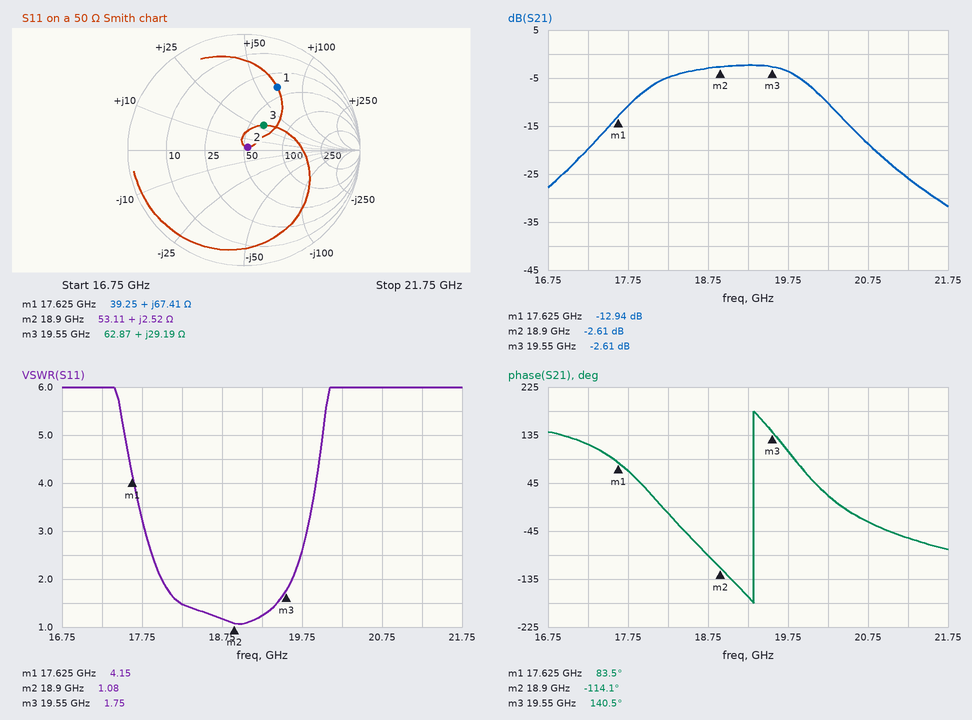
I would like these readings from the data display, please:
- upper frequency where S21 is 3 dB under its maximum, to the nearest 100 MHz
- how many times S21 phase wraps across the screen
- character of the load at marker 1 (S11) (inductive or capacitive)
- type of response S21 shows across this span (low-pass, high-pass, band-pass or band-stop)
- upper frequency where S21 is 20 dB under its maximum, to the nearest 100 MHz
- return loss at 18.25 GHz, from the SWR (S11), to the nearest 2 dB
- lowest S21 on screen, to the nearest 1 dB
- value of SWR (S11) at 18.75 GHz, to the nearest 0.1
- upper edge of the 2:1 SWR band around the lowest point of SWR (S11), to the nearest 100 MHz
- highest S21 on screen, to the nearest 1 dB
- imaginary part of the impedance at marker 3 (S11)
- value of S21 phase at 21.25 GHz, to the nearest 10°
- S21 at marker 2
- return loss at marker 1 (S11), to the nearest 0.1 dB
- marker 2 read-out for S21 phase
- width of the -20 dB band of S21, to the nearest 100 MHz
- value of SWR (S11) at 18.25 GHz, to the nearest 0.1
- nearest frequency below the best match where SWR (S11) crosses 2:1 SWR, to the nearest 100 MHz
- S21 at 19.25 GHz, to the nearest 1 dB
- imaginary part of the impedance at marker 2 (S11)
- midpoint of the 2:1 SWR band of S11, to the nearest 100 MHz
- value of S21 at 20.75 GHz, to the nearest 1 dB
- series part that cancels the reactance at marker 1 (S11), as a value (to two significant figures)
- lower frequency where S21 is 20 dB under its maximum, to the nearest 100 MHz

19.9 GHz
1
inductive
band-pass
21.0 GHz
14 dB
-32 dB
1.2
19.6 GHz
-2 dB
+29.19 Ω
-60°
-2.61 dB
4.3 dB
-114.1°
3.9 GHz
1.5
18.0 GHz
-2 dB
+2.52 Ω
18.8 GHz
-19 dB
130 fF
17.1 GHz
